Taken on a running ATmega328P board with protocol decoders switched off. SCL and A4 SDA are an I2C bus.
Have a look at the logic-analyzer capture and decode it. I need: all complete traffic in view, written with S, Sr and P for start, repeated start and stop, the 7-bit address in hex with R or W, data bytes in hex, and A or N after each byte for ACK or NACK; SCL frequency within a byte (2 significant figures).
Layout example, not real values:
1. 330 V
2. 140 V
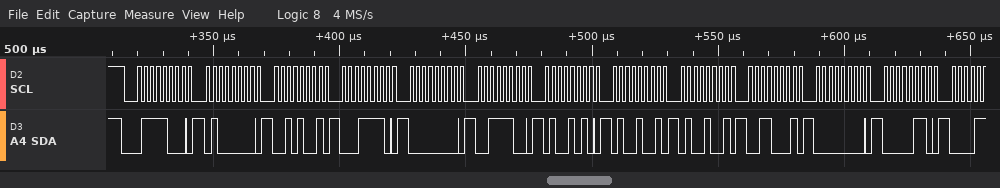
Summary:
1. S 3CW A 40 A 29 A 1E A 00 A 3C A 4A A 49 A 49 A 31 A 00 A 06 A
2. 400 kHz
